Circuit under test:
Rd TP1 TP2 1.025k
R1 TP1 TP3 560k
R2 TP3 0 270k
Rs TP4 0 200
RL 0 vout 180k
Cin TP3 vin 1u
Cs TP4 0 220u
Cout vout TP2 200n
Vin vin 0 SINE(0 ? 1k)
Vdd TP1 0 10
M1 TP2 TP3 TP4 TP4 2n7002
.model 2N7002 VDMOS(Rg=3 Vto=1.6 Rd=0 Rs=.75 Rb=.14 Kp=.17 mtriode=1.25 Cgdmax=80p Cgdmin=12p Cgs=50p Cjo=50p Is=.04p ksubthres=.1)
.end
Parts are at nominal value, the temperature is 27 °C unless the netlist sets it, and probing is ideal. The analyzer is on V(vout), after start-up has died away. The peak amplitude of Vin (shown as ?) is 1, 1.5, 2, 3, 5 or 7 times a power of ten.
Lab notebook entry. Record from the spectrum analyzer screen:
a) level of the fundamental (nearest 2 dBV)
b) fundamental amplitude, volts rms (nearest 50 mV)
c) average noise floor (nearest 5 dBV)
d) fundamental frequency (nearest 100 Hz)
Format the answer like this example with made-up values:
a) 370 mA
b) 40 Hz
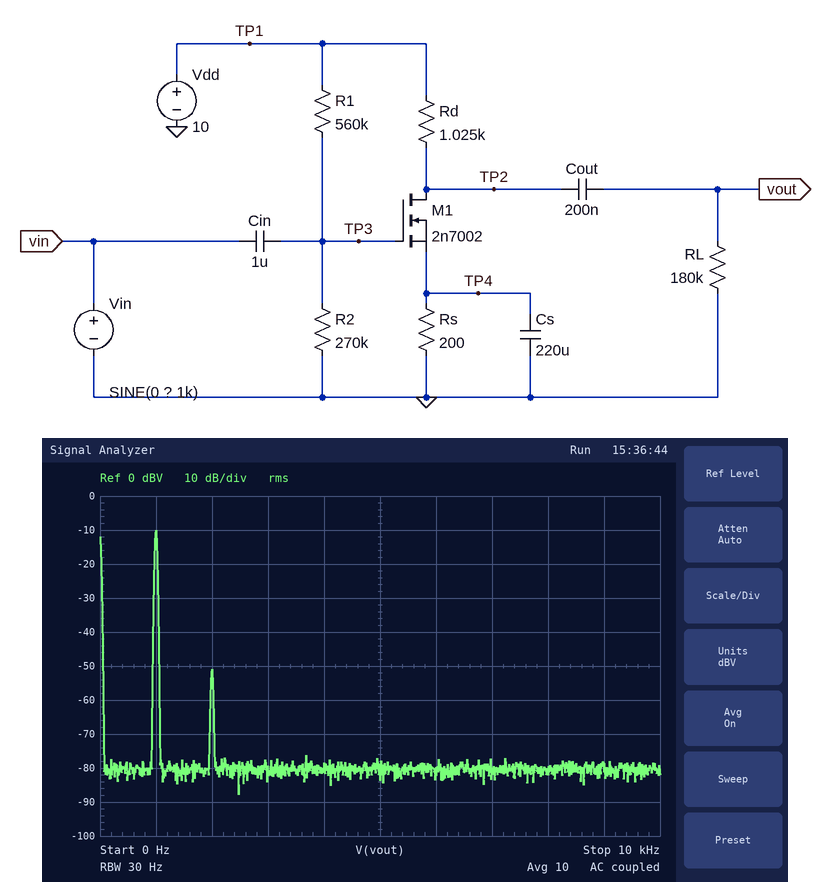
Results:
a) -10 dBV
b) 300 mV
c) -80 dBV
d) 1.0 kHz
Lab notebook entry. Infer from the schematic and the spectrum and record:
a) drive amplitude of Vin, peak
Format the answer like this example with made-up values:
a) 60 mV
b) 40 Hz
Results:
a) 10 mV
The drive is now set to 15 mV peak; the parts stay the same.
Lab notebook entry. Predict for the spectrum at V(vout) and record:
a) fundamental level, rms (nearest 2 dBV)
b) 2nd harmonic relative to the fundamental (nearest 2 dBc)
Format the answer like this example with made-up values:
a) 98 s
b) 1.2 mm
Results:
a) -6 dBV
b) -38 dBc
